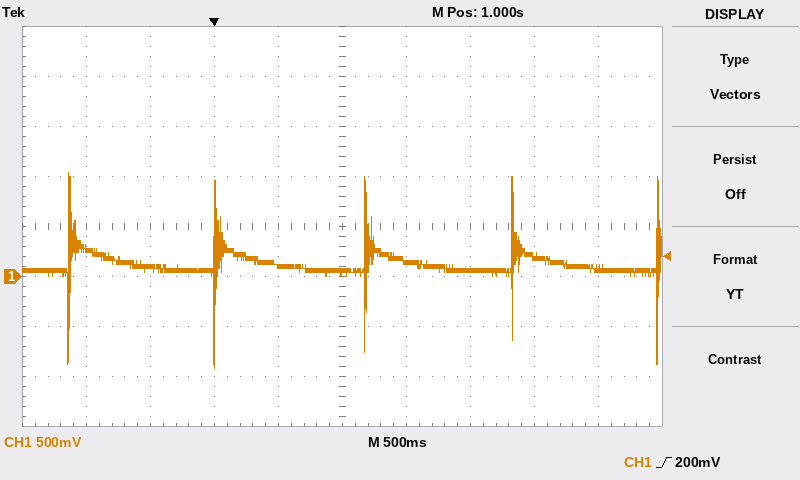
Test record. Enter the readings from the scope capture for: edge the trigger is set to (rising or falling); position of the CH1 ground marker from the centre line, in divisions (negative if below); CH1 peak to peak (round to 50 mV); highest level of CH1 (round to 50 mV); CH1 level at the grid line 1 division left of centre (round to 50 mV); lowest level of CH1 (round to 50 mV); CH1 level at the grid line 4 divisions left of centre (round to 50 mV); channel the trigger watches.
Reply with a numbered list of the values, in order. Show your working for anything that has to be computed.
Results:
1. rising
2. -1.0 div
3. 1.05 V − (-900 mV) = 1.95 V
4. 1.05 V
5. 100 mV
6. -900 mV
7. 300 mV
8. CH1
